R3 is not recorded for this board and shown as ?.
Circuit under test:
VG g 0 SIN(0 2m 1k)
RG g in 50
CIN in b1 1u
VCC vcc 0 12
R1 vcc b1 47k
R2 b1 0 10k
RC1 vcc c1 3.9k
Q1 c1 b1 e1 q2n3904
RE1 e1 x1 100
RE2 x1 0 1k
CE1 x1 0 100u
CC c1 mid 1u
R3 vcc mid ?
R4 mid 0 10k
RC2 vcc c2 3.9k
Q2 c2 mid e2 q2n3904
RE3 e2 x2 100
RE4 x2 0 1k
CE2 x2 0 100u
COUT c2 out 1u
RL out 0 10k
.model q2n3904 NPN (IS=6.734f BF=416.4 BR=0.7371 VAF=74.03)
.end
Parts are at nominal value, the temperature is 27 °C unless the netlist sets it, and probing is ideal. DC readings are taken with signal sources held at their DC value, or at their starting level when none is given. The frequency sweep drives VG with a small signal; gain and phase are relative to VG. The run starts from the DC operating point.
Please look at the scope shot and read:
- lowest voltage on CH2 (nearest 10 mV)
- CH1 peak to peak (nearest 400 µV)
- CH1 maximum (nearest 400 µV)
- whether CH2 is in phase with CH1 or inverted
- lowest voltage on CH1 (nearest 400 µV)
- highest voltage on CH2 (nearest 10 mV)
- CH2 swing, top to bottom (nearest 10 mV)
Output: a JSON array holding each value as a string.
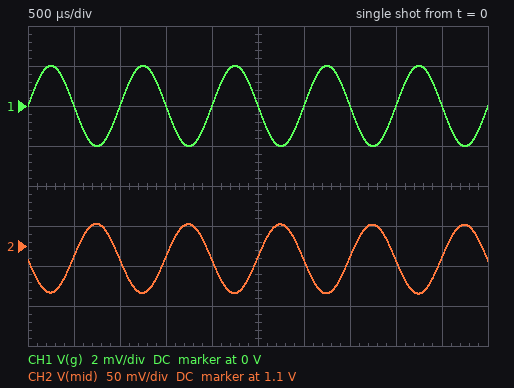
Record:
["1.04 V", "4.0 mV", "2.0 mV", "inverted", "-2.0 mV", "1.13 V", "90 mV"]
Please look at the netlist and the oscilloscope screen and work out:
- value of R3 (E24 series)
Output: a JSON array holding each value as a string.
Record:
["100 kΩ"]
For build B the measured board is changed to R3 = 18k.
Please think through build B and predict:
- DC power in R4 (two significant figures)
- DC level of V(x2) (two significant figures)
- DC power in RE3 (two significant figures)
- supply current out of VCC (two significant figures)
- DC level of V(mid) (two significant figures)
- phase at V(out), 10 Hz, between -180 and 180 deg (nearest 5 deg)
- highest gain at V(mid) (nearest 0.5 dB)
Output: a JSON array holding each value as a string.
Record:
["1.2 mW", "2.5 V", "620 µW", "4.3 mA", "3.4 V", "-45 deg", "-0.5 dB"]
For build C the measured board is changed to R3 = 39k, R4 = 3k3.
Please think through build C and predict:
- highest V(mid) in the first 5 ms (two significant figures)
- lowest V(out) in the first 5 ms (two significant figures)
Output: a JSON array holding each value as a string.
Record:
["960 mV", "-470 mV"]
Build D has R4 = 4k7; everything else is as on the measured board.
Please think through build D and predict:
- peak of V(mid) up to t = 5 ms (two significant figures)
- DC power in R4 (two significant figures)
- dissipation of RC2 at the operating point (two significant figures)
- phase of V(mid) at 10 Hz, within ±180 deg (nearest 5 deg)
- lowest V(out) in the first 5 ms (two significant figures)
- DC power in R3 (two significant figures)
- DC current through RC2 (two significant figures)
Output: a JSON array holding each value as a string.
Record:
["570 mV", "62 µW", "170 nW", "-10 deg", "-49 mV", "1.3 mW", "6.5 µA"]
